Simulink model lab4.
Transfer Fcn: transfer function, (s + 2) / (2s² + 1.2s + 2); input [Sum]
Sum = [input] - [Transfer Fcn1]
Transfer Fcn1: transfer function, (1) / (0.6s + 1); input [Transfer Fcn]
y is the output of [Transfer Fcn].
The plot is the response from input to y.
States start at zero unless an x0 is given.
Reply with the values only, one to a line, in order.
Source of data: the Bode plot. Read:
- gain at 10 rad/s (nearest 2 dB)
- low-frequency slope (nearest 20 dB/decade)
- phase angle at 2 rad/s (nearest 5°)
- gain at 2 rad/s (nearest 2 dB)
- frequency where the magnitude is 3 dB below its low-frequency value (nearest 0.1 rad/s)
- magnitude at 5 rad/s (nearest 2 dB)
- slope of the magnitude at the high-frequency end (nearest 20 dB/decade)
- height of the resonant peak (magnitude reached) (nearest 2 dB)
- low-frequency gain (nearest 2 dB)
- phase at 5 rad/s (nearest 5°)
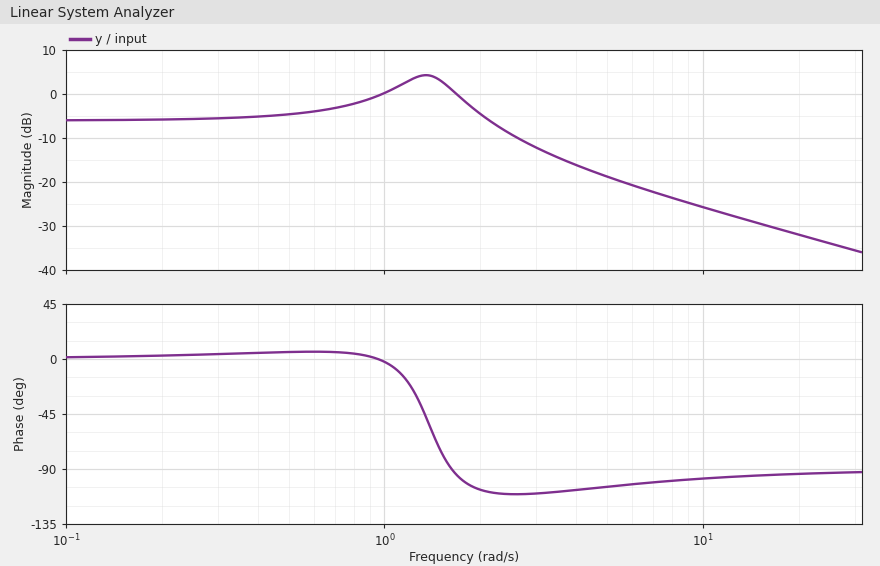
-26 dB
0 dB/decade
-105°
-4 dB
2.5 rad/s
-18 dB
-20 dB/decade
4 dB
-6 dB
-105°
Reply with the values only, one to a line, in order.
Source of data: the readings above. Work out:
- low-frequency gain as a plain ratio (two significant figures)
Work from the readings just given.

0.50
